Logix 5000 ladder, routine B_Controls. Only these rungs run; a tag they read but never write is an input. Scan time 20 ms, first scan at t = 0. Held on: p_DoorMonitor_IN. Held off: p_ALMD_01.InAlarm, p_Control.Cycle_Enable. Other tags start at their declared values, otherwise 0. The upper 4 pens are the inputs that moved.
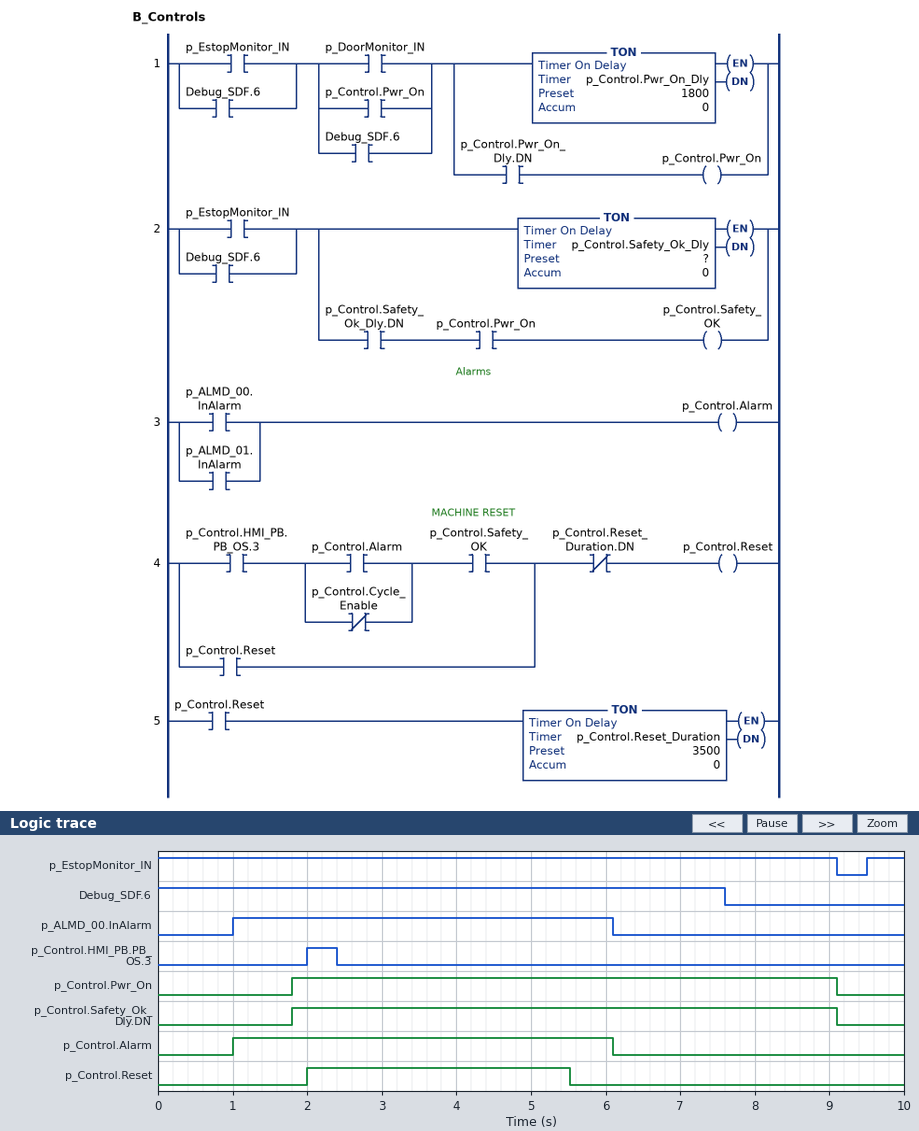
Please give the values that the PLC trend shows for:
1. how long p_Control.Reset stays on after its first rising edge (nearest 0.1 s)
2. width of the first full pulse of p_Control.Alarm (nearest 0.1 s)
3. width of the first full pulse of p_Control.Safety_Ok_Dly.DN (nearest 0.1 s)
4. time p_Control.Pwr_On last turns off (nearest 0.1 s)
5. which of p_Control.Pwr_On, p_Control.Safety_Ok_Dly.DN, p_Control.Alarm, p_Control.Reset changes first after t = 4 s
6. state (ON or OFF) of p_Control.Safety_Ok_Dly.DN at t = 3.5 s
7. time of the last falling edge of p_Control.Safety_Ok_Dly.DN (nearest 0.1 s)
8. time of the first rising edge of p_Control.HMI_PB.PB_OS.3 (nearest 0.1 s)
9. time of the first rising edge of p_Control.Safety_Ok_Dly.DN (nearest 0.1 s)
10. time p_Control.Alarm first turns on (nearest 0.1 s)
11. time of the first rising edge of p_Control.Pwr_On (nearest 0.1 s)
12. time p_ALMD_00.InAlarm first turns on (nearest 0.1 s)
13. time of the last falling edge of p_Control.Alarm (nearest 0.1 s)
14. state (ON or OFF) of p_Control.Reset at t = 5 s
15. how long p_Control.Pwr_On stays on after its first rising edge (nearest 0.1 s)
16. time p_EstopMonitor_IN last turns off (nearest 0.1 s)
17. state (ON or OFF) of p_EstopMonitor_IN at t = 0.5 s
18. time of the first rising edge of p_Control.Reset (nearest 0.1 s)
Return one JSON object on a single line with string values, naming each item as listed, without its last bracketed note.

{"how long p_Control.Reset stays on after its first rising edge": "3.5 s", "width of the first full pulse of p_Control.Alarm": "5.1 s", "width of the first full pulse of p_Control.Safety_Ok_Dly.DN": "7.3 s", "time p_Control.Pwr_On last turns off": "9.1 s", "which of p_Control.Pwr_On, p_Control.Safety_Ok_Dly.DN, p_Control.Alarm, p_Control.Reset changes first after t = 4 s": "p_Control.Reset", "state (ON or OFF) of p_Control.Safety_Ok_Dly.DN at t = 3.5 s": "ON", "time of the last falling edge of p_Control.Safety_Ok_Dly.DN": "9.1 s", "time of the first rising edge of p_Control.HMI_PB.PB_OS.3": "2.0 s", "time of the first rising edge of p_Control.Safety_Ok_Dly.DN": "1.8 s", "time p_Control.Alarm first turns on": "1.0 s", "time of the first rising edge of p_Control.Pwr_On": "1.8 s", "time p_ALMD_00.InAlarm first turns on": "1.0 s", "time of the last falling edge of p_Control.Alarm": "6.1 s", "state (ON or OFF) of p_Control.Reset at t = 5 s": "ON", "how long p_Control.Pwr_On stays on after its first rising edge": "7.3 s", "time p_EstopMonitor_IN last turns off": "9.1 s", "state (ON or OFF) of p_EstopMonitor_IN at t = 0.5 s": "ON", "time of the first rising edge of p_Control.Reset": "2.0 s"}
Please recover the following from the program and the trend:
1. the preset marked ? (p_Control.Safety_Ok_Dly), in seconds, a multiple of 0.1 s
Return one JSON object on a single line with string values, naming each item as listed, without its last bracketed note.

{"the preset marked ? (p_Control.Safety_Ok_Dly), in seconds, a multiple of 0.1 s": "1.8 s"}
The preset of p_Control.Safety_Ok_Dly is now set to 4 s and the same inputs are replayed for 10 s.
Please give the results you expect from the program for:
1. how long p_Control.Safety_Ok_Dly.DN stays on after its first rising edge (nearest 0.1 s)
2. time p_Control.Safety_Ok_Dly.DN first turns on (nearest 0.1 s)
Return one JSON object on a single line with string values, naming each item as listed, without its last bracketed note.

{"how long p_Control.Safety_Ok_Dly.DN stays on after its first rising edge": "5.1 s", "time p_Control.Safety_Ok_Dly.DN first turns on": "4.0 s"}
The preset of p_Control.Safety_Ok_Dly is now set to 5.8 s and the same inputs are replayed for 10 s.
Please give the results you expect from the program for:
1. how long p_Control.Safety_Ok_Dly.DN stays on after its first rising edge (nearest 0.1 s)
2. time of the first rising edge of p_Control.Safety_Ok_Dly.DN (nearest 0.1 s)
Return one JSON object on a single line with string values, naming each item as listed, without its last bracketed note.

{"how long p_Control.Safety_Ok_Dly.DN stays on after its first rising edge": "3.3 s", "time of the first rising edge of p_Control.Safety_Ok_Dly.DN": "5.8 s"}
